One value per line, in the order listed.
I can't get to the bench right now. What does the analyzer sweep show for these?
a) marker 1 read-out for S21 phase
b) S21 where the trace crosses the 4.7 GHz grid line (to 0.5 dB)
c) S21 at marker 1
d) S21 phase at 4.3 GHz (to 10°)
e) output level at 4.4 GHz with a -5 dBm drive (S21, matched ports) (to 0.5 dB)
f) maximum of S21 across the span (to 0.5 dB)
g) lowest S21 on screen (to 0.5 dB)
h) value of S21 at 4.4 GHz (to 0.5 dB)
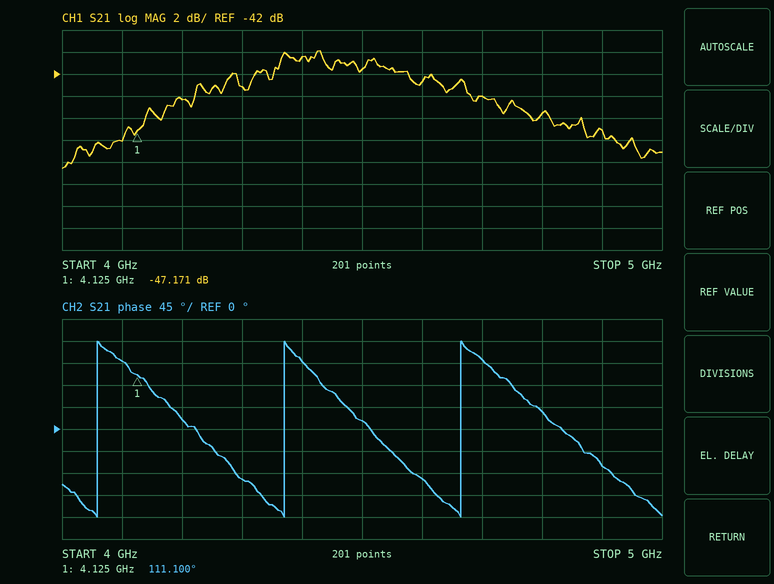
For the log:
111.100°
-44.0 dB
-47.171 dB
-100°
-45.5 dBm
-40.0 dB
-50.5 dB
-40.5 dB
